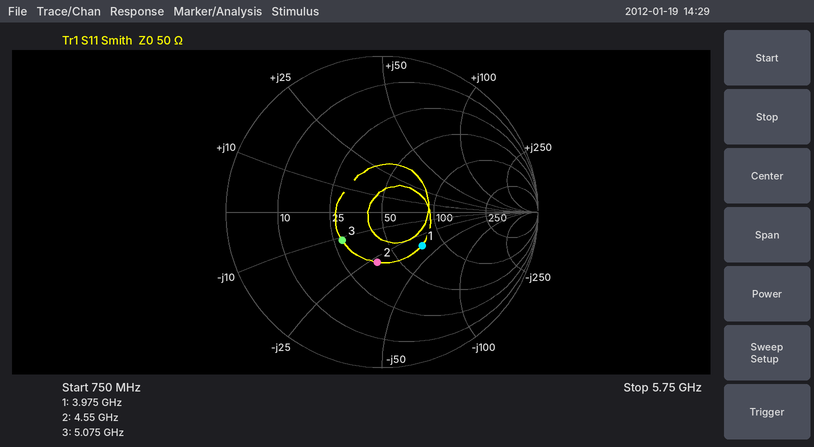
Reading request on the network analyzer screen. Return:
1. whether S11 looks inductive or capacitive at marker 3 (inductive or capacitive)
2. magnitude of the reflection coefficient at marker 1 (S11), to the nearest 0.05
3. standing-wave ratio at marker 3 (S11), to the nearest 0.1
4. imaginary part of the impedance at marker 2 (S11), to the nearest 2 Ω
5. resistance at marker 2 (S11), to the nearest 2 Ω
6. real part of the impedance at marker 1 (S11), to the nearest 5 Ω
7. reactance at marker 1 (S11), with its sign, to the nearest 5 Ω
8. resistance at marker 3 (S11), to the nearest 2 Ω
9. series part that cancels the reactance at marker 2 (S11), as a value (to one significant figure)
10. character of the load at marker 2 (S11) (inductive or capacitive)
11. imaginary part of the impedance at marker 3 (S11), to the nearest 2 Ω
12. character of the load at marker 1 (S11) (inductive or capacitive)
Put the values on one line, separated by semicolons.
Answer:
capacitive; 0.35; 1.9; -28 Ω; 38 Ω; 75 Ω; -35 Ω; 28 Ω; 1.0 nH; capacitive; -12 Ω; capacitive
